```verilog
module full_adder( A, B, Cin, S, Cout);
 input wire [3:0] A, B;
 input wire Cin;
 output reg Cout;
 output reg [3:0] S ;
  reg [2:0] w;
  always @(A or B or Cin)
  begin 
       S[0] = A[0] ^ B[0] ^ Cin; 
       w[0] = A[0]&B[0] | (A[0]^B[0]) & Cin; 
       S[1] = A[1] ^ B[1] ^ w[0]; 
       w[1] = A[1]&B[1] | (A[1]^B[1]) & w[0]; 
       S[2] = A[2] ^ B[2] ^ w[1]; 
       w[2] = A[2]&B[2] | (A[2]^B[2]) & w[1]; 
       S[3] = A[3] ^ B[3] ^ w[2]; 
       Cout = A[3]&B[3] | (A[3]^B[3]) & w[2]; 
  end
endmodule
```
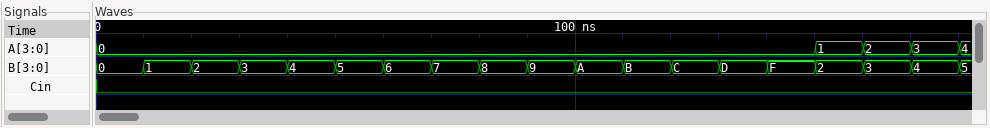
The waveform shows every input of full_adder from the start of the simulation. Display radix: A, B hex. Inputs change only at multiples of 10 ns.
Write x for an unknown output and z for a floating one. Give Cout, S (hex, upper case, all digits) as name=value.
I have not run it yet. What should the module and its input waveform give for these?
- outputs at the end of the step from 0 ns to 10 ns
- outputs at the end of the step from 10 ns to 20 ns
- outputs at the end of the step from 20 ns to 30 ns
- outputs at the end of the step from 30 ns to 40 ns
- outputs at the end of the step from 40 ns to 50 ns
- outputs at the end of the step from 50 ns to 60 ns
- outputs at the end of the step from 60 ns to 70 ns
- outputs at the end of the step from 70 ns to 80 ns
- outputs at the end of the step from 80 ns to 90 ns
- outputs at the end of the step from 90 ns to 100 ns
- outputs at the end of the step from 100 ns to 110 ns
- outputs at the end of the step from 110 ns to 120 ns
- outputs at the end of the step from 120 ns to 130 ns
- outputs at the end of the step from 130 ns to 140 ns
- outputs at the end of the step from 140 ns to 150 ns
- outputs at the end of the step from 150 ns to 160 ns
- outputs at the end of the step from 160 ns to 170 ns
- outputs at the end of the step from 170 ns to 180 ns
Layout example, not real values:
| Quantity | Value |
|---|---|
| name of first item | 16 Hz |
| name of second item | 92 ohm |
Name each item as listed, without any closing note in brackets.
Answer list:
| Quantity | Value |
|---|---|
| outputs at the end of the step from 0 ns to 10 ns | Cout=0, S=0 |
| outputs at the end of the step from 10 ns to 20 ns | Cout=0, S=1 |
| outputs at the end of the step from 20 ns to 30 ns | Cout=0, S=2 |
| outputs at the end of the step from 30 ns to 40 ns | Cout=0, S=3 |
| outputs at the end of the step from 40 ns to 50 ns | Cout=0, S=4 |
| outputs at the end of the step from 50 ns to 60 ns | Cout=0, S=5 |
| outputs at the end of the step from 60 ns to 70 ns | Cout=0, S=6 |
| outputs at the end of the step from 70 ns to 80 ns | Cout=0, S=7 |
| outputs at the end of the step from 80 ns to 90 ns | Cout=0, S=8 |
| outputs at the end of the step from 90 ns to 100 ns | Cout=0, S=9 |
| outputs at the end of the step from 100 ns to 110 ns | Cout=0, S=A |
| outputs at the end of the step from 110 ns to 120 ns | Cout=0, S=B |
| outputs at the end of the step from 120 ns to 130 ns | Cout=0, S=C |
| outputs at the end of the step from 130 ns to 140 ns | Cout=0, S=D |
| outputs at the end of the step from 140 ns to 150 ns | Cout=0, S=F |
| outputs at the end of the step from 150 ns to 160 ns | Cout=0, S=3 |
| outputs at the end of the step from 160 ns to 170 ns | Cout=0, S=5 |
| outputs at the end of the step from 170 ns to 180 ns | Cout=0, S=7 |
